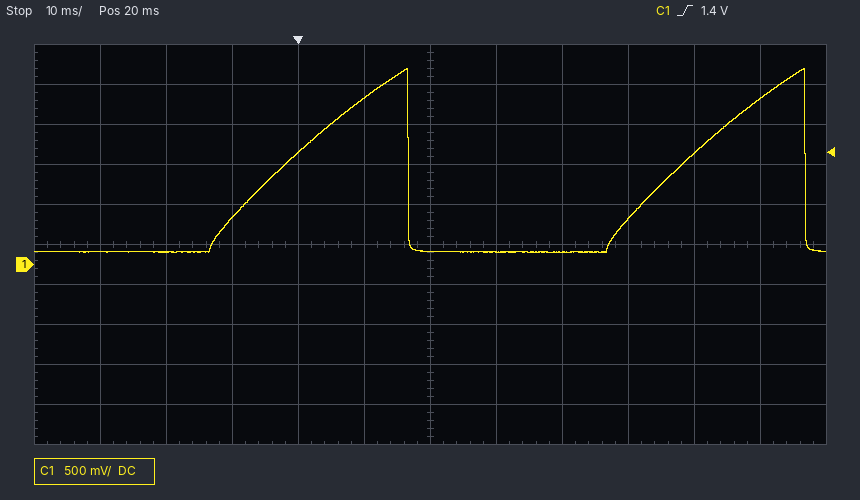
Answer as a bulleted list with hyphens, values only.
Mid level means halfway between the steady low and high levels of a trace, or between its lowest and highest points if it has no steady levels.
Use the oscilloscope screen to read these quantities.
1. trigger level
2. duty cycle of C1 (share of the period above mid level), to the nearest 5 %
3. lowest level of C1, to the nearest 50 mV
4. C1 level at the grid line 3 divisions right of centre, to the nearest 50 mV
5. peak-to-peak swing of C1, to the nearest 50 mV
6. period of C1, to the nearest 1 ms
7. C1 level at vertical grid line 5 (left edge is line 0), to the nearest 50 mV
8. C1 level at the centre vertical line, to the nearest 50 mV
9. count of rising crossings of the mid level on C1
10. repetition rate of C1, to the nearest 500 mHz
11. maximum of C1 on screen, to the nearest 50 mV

- 1.4 V
- 30 %
- 150 mV
- 550 mV
- 2.30 V
- 60 ms
- 2.10 V
- 150 mV
- 2
- 16.5 Hz
- 2.45 V
